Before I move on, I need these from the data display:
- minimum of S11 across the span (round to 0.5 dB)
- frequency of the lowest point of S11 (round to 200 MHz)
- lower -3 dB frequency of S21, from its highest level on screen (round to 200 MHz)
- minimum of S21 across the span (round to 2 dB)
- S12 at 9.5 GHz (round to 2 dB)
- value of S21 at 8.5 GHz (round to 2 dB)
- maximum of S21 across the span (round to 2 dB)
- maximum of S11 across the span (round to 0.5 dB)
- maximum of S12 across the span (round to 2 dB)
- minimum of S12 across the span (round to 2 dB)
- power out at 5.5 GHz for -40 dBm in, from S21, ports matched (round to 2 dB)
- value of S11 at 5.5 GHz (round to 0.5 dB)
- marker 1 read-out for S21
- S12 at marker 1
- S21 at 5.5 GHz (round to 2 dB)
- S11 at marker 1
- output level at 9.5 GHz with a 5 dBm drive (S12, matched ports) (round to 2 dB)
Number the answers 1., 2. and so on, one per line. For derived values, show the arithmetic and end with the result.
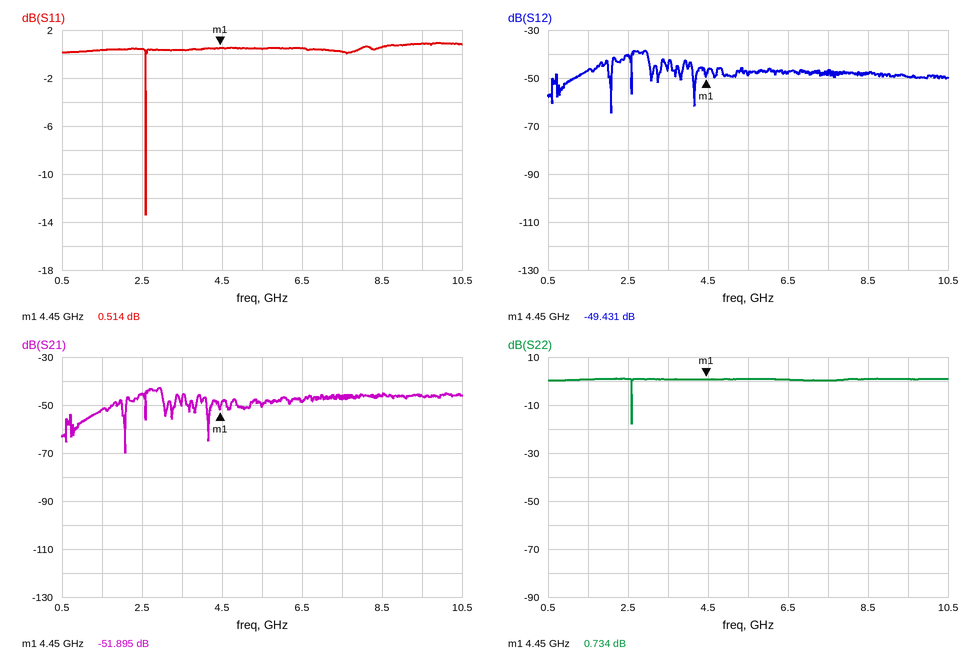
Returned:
1. -13.5 dB
2. 2.6 GHz
3. 2.6 GHz
4. -70 dB
5. -50 dB
6. -46 dB
7. -42 dB
8. 1.0 dB
9. -38 dB
10. -64 dB
11. -40 dBm + (-50 dB) = -90 dBm
12. 0.5 dB
13. -51.895 dB
14. -49.431 dB
15. -50 dB
16. 0.514 dB
17. 5 dBm + (-50 dB) = -44 dBm
